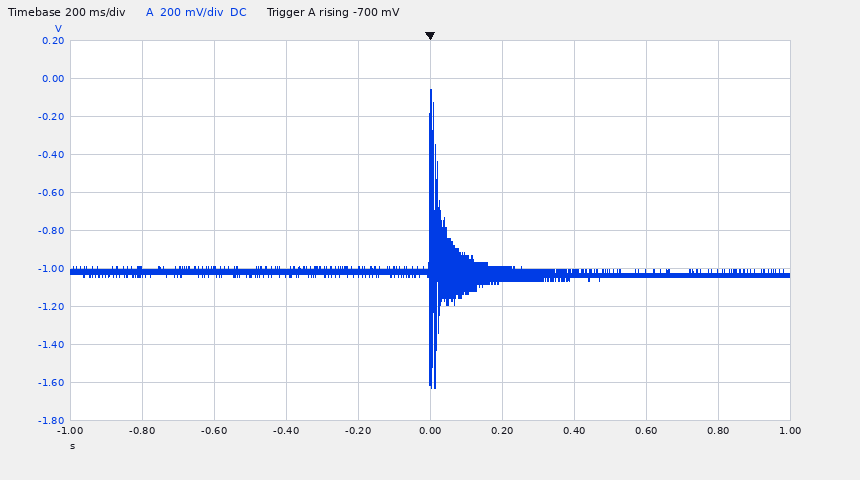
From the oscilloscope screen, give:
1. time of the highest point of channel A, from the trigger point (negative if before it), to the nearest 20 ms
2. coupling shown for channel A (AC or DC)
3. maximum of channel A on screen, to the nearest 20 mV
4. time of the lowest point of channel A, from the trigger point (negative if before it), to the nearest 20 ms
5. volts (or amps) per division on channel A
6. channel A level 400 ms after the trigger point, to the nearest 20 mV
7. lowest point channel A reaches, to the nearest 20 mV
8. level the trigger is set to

0 ms
DC
-60 mV
0 ms
200 mV
-1.02 V
-1.62 V
-700 mV
